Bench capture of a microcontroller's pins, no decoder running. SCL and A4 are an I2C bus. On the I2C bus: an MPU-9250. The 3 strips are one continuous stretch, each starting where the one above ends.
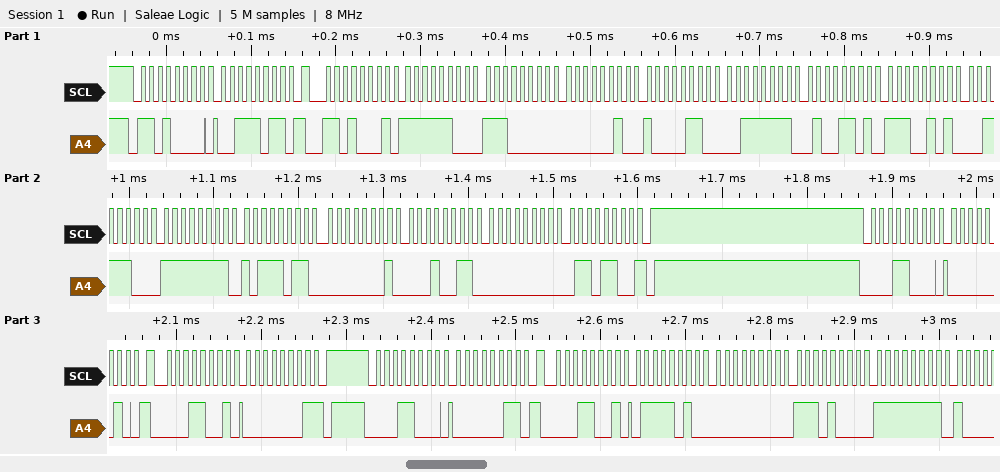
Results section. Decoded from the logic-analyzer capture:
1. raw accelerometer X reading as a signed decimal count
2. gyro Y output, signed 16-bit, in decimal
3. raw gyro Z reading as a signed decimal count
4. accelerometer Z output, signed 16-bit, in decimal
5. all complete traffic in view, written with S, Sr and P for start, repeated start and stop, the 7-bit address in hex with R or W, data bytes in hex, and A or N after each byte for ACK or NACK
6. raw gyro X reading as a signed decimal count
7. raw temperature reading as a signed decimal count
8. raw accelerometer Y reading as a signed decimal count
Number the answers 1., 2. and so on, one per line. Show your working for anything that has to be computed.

1. 0xFCE0 = -800
2. 0x0113 = 275
3. 0x006C = 108
4. 0x3F4D = 16205
5. S 68W A 3B A Sr 68R A FC A E0 A 02 A 86 A 3F A 4D A E5 A 3C A FF A BB A 01 A 13 A 00 A 6C N P S 0CW A 02 A Sr 0CR A 01 N P S 0CW A 03 A Sr 0CR A 7A A 00 A E8 A FF A
6. 0xFFBB = -69
7. 0xE53C = -6852
8. 0x0286 = 646
